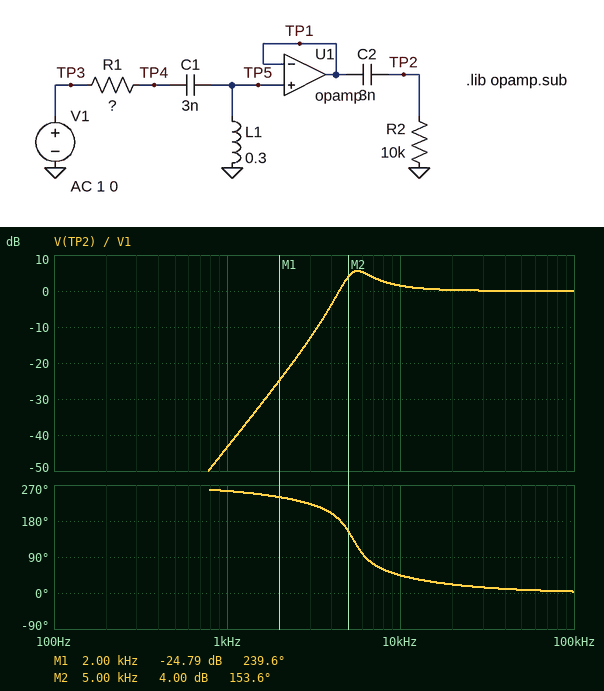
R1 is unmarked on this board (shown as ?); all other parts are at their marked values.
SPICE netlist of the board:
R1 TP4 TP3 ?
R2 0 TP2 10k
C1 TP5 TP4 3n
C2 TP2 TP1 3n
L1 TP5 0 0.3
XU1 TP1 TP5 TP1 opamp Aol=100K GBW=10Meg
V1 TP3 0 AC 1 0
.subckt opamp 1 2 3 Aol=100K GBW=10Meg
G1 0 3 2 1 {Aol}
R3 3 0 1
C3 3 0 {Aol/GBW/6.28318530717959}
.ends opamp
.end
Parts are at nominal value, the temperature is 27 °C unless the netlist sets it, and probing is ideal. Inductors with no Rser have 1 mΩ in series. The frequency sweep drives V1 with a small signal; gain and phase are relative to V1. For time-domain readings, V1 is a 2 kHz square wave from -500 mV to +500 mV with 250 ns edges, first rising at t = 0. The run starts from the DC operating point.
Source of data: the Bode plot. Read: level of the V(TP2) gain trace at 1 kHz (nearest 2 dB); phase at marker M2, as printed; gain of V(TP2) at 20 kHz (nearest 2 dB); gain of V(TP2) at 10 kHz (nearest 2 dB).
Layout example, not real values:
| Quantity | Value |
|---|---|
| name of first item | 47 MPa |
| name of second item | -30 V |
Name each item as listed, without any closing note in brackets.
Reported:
| Quantity | Value |
|---|---|
| level of the V(TP2) gain trace at 1 kHz | -44 dB |
| phase at marker M2, as printed | 153.6 deg |
| gain of V(TP2) at 20 kHz | 0 dB |
| gain of V(TP2) at 10 kHz | 2 dB |
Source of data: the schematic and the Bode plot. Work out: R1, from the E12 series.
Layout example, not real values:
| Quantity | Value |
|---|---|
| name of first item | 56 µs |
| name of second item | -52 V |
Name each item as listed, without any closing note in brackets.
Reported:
| Quantity | Value |
|---|---|
| R1, from the E12 series | 3.9 kΩ |
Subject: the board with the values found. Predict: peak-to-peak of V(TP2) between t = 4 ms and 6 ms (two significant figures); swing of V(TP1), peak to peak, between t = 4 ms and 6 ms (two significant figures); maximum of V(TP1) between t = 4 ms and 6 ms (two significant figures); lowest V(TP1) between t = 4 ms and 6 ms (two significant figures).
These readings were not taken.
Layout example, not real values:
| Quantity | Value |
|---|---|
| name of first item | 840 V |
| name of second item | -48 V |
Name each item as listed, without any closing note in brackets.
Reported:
| Quantity | Value |
|---|---|
| peak-to-peak of V(TP2) between t = 4 ms and 6 ms | 2.3 V |
| swing of V(TP1), peak to peak, between t = 4 ms and 6 ms | 2.1 V |
| maximum of V(TP1) between t = 4 ms and 6 ms | 1.1 V |
| lowest V(TP1) between t = 4 ms and 6 ms | -1.1 V |
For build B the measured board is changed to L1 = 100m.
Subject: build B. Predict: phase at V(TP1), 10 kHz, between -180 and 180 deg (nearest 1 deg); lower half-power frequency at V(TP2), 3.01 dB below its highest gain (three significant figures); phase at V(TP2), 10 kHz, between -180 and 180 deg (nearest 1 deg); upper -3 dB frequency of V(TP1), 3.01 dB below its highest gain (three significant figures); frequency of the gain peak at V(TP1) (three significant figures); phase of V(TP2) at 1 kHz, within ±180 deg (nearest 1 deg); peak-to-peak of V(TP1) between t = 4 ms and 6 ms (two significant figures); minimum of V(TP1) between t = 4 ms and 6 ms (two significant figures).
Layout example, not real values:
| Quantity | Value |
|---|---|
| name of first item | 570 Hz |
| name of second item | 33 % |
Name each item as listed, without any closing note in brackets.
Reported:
| Quantity | Value |
|---|---|
| phase at V(TP1), 10 kHz, between -180 and 180 deg | 76 deg |
| lower half-power frequency at V(TP2), 3.01 dB below its highest gain | 8.01 kHz |
| phase at V(TP2), 10 kHz, between -180 and 180 deg | 104 deg |
| upper -3 dB frequency of V(TP1), 3.01 dB below its highest gain | 24.9 kHz |
| frequency of the gain peak at V(TP1) | 10.5 kHz |
| phase of V(TP2) at 1 kHz, within ±180 deg | -105 deg |
| peak-to-peak of V(TP1) between t = 4 ms and 6 ms | 2.0 V |
| minimum of V(TP1) between t = 4 ms and 6 ms | -990 mV |
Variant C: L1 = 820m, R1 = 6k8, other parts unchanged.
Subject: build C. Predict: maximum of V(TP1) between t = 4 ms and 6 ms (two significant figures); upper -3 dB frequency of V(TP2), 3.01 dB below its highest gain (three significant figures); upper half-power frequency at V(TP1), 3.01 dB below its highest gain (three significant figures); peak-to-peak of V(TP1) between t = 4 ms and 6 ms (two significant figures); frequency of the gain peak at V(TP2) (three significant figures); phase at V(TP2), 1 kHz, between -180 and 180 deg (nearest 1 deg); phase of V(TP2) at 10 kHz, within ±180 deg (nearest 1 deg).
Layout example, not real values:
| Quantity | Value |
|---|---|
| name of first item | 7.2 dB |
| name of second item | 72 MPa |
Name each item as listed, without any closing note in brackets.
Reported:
| Quantity | Value |
|---|---|
| maximum of V(TP1) between t = 4 ms and 6 ms | 780 mV |
| upper -3 dB frequency of V(TP2), 3.01 dB below its highest gain | 3.24 MHz |
| upper half-power frequency at V(TP1), 3.01 dB below its highest gain | 4.48 kHz |
| peak-to-peak of V(TP1) between t = 4 ms and 6 ms | 1.6 V |
| frequency of the gain peak at V(TP2) | 3.49 kHz |
| phase at V(TP2), 1 kHz, between -180 and 180 deg | -109 deg |
| phase of V(TP2) at 10 kHz, within ±180 deg | 36 deg |
